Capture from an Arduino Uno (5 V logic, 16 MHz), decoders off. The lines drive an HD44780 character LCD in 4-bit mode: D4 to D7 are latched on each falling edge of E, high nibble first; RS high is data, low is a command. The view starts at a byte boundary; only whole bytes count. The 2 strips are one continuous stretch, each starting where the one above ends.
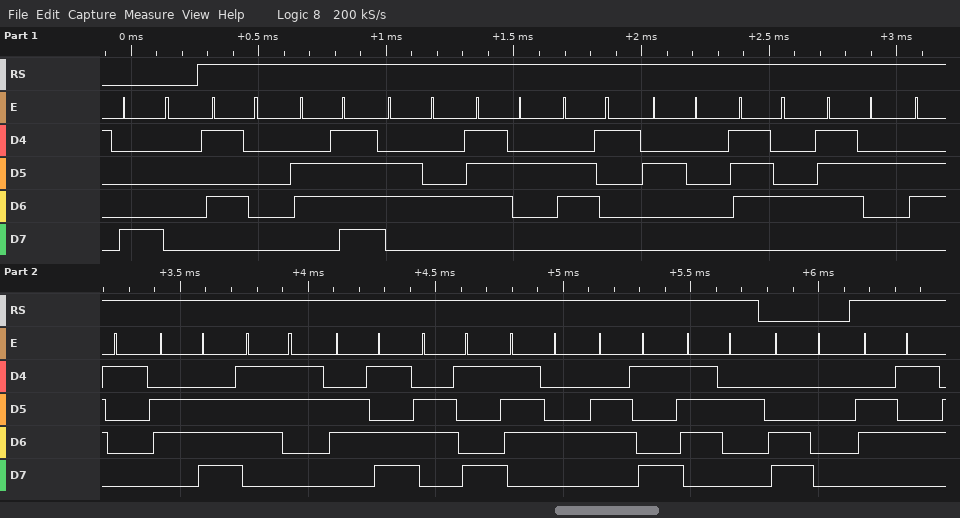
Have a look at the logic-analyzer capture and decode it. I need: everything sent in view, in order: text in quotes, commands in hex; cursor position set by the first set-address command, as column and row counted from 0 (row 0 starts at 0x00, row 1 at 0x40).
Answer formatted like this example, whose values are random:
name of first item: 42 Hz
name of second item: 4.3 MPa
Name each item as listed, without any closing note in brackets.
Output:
everything sent in view, in order: text in quotes, commands in hex: 0x80 "Podra transmitir" 0xC0 "e"
cursor position set by the first set-address command, as column and row counted from 0: column 0, row 0
